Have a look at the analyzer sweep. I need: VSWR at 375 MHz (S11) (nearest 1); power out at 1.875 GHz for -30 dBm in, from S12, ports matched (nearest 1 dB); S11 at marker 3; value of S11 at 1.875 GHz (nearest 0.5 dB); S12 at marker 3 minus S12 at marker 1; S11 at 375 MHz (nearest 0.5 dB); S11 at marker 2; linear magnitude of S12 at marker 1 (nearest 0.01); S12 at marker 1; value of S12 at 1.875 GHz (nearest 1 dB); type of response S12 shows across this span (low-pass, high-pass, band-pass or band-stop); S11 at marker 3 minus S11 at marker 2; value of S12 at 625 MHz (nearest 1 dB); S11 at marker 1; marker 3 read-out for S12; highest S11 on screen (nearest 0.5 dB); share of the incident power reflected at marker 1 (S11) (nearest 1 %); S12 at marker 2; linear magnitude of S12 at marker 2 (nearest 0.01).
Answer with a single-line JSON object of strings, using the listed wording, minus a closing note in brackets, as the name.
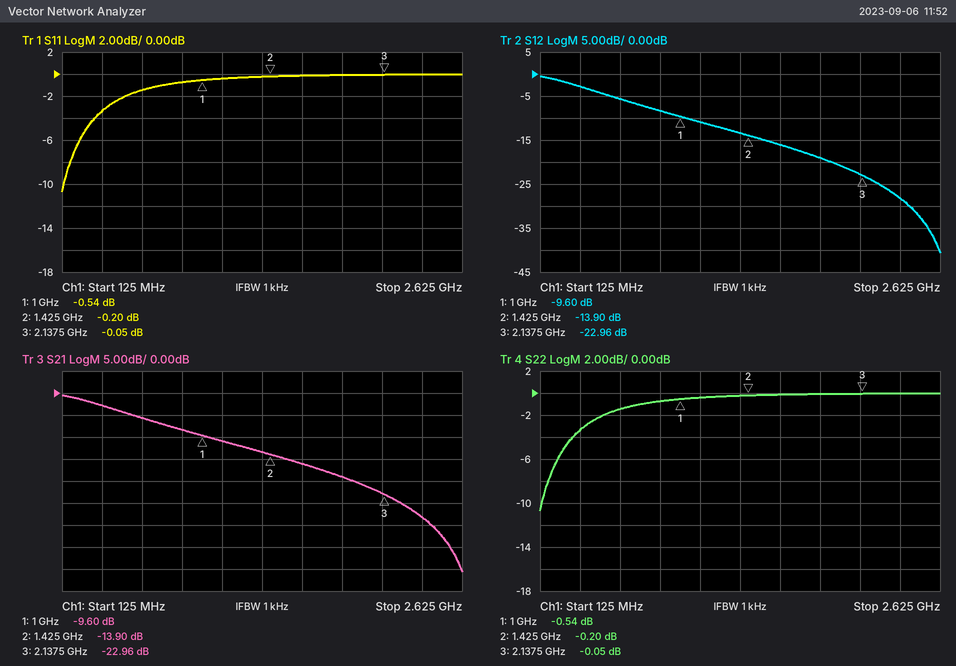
{"VSWR at 375 MHz (S11)": "5", "power out at 1.875 GHz for -30 dBm in, from S12, ports matched": "-49 dBm", "S11 at marker 3": "-0.05 dB", "value of S11 at 1.875 GHz": "0.0 dB", "S12 at marker 3 minus S12 at marker 1": "-13.36 dB", "S11 at 375 MHz": "-3.5 dB", "S11 at marker 2": "-0.20 dB", "linear magnitude of S12 at marker 1": "0.33", "S12 at marker 1": "-9.60 dB", "value of S12 at 1.875 GHz": "-19 dB", "type of response S12 shows across this span": "low-pass", "S11 at marker 3 minus S11 at marker 2": "0.15 dB", "value of S12 at 625 MHz": "-6 dB", "S11 at marker 1": "-0.54 dB", "marker 3 read-out for S12": "-22.96 dB", "highest S11 on screen": "0.0 dB", "share of the incident power reflected at marker 1 (S11)": "88 %", "S12 at marker 2": "-13.90 dB", "linear magnitude of S12 at marker 2": "0.20"}
